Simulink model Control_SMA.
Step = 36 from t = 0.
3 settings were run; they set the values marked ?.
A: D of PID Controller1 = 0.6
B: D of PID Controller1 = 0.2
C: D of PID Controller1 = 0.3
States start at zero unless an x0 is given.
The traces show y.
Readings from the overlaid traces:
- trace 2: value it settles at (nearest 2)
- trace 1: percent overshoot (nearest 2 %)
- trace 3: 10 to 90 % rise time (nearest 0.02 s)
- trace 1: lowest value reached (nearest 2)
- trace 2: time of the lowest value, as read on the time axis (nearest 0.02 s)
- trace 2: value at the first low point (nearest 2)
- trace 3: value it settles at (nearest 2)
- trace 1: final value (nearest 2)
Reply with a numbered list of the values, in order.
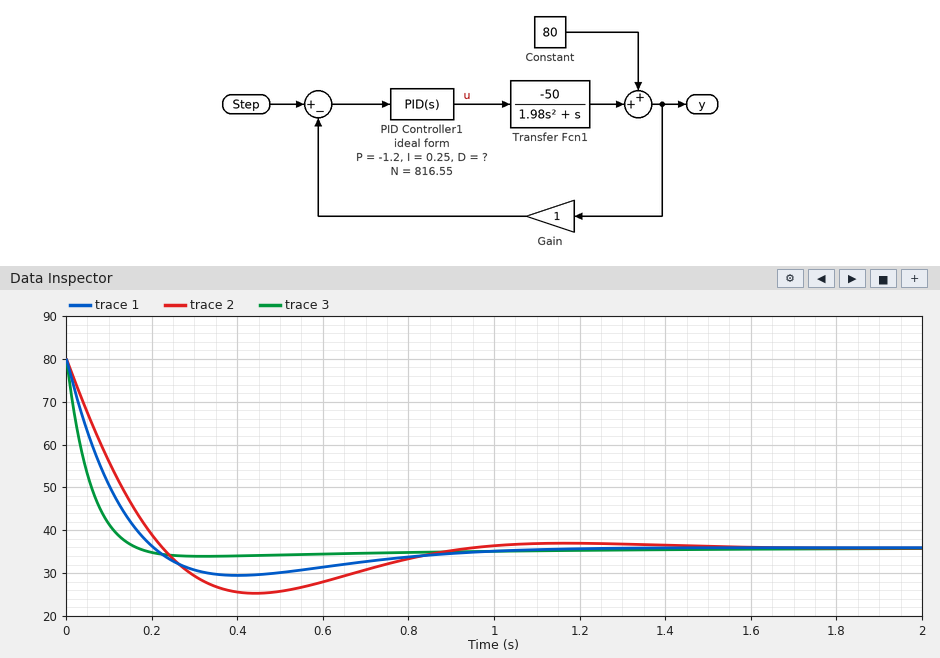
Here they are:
1. 36
2. 14 %
3. 0.10 s
4. 30
5. 0.44 s
6. 26
7. 36
8. 36
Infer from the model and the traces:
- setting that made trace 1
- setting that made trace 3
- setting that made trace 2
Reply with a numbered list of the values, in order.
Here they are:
1. C
2. A
3. B
